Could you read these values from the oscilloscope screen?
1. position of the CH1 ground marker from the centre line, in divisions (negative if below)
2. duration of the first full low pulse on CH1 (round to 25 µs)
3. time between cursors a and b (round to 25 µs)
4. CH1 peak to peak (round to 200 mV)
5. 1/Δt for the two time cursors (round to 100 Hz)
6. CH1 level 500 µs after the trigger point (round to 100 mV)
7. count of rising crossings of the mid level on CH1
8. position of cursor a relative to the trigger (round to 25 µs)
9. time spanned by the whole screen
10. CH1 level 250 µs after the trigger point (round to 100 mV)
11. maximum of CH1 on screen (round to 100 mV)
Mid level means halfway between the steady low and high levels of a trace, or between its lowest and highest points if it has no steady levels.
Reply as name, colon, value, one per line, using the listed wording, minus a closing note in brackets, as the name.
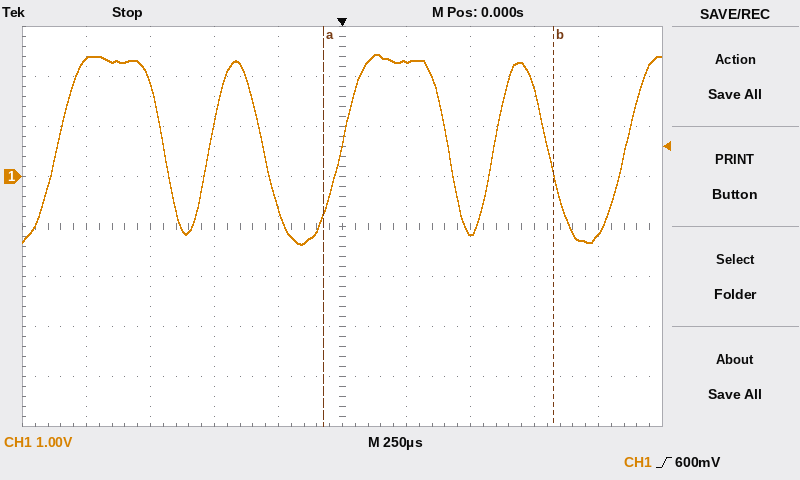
position of the CH1 ground marker from the centre line, in divisions: +1.0 div
duration of the first full low pulse on CH1: 175 µs
time between cursors a and b: 900 µs
CH1 peak to peak: 3.8 V
1/Δt for the two time cursors: 1.1 kHz
CH1 level 500 µs after the trigger point: -1.1 V
count of rising crossings of the mid level on CH1: 5
position of cursor a relative to the trigger: -75 µs
time spanned by the whole screen: 2.5 ms
CH1 level 250 µs after the trigger point: 2.3 V
maximum of CH1 on screen: 2.4 V
